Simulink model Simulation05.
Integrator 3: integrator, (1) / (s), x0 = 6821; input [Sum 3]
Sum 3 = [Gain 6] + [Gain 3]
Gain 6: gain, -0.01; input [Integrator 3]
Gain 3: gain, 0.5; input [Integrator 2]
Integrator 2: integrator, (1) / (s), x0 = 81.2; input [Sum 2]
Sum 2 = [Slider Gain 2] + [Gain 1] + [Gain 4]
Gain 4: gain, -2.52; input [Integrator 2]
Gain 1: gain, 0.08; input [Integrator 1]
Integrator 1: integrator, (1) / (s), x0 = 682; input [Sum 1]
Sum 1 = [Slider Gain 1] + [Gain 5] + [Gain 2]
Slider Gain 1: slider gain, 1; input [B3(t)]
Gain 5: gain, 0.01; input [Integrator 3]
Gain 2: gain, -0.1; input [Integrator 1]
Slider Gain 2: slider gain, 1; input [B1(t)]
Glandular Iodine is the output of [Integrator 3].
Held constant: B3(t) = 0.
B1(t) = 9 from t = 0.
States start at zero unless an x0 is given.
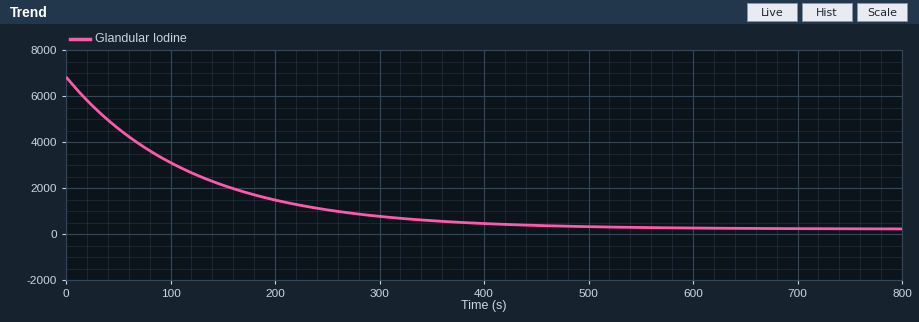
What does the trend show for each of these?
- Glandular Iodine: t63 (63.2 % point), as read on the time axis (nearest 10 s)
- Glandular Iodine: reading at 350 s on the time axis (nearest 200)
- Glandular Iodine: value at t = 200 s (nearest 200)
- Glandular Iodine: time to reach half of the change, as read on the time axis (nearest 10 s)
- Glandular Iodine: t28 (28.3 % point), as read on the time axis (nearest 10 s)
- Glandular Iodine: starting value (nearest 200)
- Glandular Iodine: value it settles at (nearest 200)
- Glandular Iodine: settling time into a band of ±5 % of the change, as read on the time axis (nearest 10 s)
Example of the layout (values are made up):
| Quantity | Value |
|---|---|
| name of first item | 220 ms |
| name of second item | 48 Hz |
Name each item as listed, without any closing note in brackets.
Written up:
| Quantity | Value |
|---|---|
| Glandular Iodine: t63 (63.2 % point), as read on the time axis | 120 s |
| Glandular Iodine: reading at 350 s on the time axis | 600 |
| Glandular Iodine: value at t = 200 s | 1400 |
| Glandular Iodine: time to reach half of the change, as read on the time axis | 80 s |
| Glandular Iodine: t28 (28.3 % point), as read on the time axis | 40 s |
| Glandular Iodine: starting value | 6800 |
| Glandular Iodine: value it settles at | 200 |
| Glandular Iodine: settling time into a band of ±5 % of the change, as read on the time axis | 360 s |
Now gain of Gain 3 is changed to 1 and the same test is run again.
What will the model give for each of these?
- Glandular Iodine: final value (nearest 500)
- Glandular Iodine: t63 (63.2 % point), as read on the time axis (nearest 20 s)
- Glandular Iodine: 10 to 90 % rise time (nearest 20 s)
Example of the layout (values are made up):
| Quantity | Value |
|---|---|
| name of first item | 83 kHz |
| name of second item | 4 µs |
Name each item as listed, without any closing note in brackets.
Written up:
| Quantity | Value |
|---|---|
| Glandular Iodine: final value | 500 |
| Glandular Iodine: t63 (63.2 % point), as read on the time axis | 160 s |
| Glandular Iodine: 10 to 90 % rise time | 340 s |
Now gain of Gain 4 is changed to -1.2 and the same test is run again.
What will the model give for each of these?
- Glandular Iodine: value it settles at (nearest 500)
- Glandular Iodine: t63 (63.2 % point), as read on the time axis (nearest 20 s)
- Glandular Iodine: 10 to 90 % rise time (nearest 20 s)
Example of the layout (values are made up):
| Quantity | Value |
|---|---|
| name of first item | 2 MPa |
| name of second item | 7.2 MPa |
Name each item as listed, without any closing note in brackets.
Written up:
| Quantity | Value |
|---|---|
| Glandular Iodine: value it settles at | 500 |
| Glandular Iodine: t63 (63.2 % point), as read on the time axis | 160 s |
| Glandular Iodine: 10 to 90 % rise time | 340 s |
